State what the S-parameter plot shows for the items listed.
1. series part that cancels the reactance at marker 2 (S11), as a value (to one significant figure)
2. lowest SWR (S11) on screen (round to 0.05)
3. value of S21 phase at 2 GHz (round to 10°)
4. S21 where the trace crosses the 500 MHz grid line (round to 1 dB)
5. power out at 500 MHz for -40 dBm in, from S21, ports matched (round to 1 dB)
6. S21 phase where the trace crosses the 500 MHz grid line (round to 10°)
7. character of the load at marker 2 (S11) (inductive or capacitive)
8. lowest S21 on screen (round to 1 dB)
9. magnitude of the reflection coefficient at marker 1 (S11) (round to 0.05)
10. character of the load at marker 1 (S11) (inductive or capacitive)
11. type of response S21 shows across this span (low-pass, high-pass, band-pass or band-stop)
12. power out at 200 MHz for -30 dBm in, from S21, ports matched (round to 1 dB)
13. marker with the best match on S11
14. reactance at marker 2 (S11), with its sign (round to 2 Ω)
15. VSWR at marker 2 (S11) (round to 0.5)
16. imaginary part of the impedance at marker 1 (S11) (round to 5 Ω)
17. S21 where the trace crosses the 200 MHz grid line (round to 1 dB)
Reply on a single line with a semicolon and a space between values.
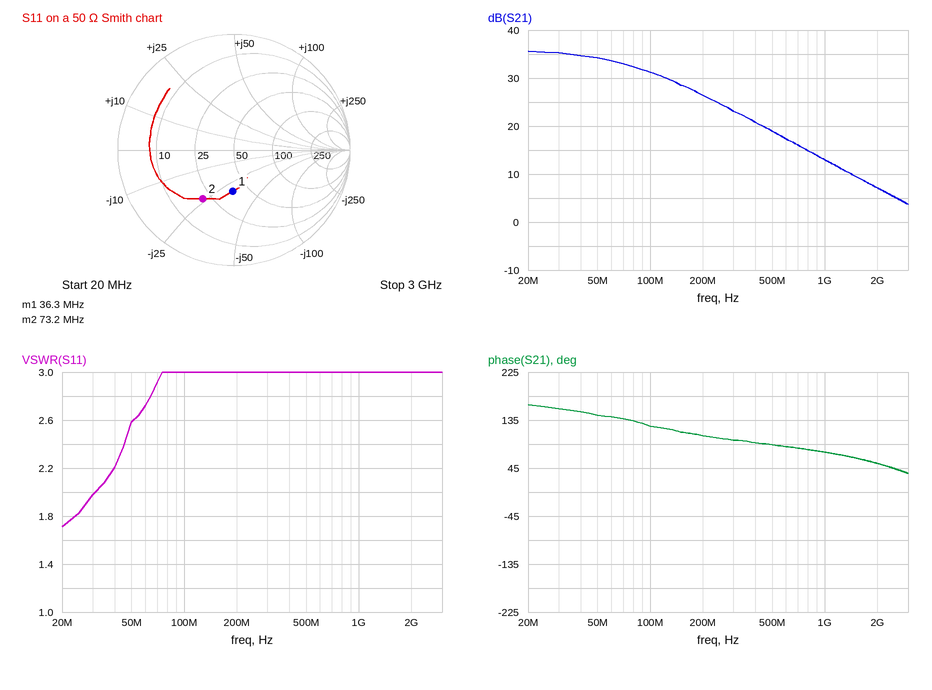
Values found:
50 nH; 1.70; 50°; 19 dB; -21 dBm; 90°; capacitive; 4 dB; 0.35; capacitive; low-pass; -4 dBm; marker 1; -24 Ω; 3.0; -30 Ω; 26 dB
